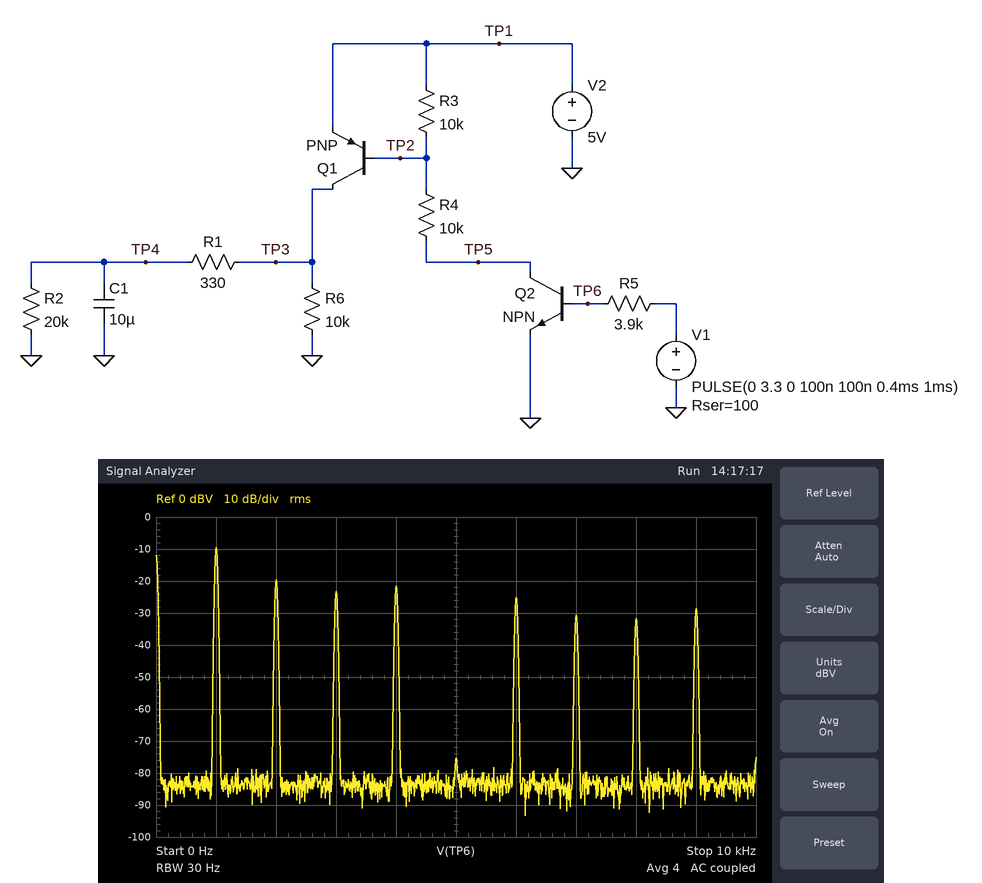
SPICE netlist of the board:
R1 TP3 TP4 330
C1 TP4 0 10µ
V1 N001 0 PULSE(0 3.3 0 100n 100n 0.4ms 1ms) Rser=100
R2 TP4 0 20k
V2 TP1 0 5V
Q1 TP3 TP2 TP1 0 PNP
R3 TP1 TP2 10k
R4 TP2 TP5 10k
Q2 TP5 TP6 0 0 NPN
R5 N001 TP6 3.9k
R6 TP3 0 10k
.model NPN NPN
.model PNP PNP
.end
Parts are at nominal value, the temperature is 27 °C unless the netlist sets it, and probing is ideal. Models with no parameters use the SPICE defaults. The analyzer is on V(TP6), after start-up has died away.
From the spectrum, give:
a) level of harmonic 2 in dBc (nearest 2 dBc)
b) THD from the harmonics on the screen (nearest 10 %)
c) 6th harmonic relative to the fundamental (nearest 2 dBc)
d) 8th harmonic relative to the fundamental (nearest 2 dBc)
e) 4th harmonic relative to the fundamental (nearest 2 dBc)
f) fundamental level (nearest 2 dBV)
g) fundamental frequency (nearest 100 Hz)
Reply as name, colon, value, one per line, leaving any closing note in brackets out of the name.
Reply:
level of harmonic 2 in dBc: -10 dBc
THD from the harmonics on the screen: 50 %
6th harmonic relative to the fundamental: -16 dBc
8th harmonic relative to the fundamental: -22 dBc
4th harmonic relative to the fundamental: -12 dBc
fundamental level: -10 dBV
fundamental frequency: 1.0 kHz
